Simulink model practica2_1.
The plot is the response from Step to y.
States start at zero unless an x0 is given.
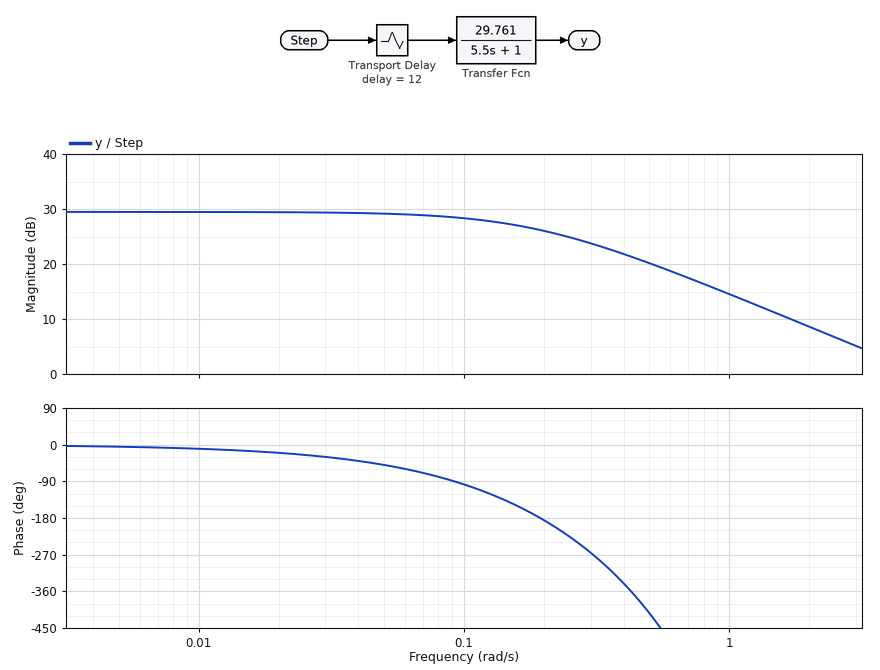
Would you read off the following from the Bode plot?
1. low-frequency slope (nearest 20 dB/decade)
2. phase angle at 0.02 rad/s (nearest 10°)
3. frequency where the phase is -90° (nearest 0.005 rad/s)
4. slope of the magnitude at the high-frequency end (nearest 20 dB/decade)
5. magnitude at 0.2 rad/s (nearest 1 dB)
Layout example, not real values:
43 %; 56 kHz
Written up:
0 dB/decade; -20°; 0.090 rad/s; -20 dB/decade; 26 dB
